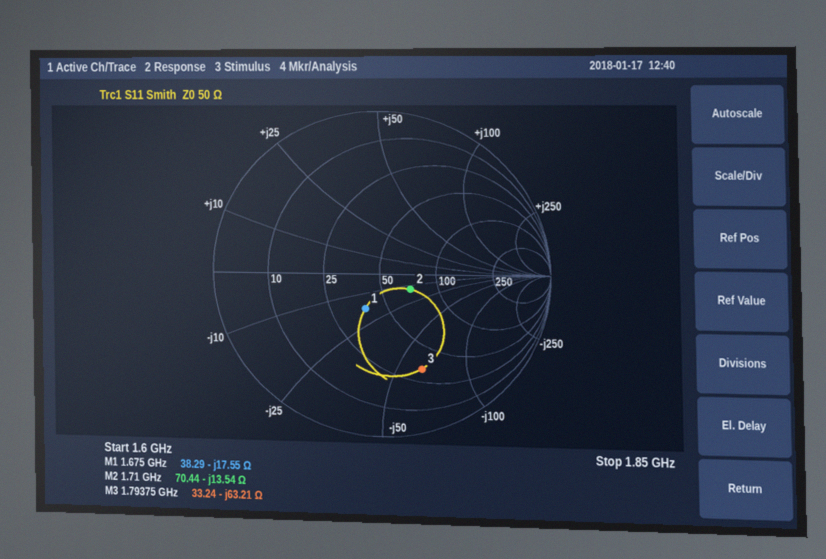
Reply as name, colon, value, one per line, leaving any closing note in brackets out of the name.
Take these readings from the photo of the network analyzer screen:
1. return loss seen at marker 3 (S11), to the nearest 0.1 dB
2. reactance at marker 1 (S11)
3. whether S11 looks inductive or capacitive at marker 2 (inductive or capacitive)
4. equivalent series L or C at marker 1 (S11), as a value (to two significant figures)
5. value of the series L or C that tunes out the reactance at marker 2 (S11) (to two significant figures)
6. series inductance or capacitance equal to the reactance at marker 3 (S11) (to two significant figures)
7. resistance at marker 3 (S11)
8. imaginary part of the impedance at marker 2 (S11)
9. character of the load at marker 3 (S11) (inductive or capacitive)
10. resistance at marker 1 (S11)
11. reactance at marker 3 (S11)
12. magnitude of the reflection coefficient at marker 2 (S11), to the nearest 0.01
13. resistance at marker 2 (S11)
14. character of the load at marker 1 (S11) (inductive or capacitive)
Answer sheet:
return loss seen at marker 3 (S11), to the nearest 0.1 dB: 4.1 dB
reactance at marker 1: -17.55 Ω
whether S11 looks inductive or capacitive at marker 2: capacitive
equivalent series L or C at marker 1 (S11), as a value: 5.4 pF
value of the series L or C that tunes out the reactance at marker 2 (S11): 1.3 nH
series inductance or capacitance equal to the reactance at marker 3 (S11): 1.4 pF
resistance at marker 3: 33.24 Ω
imaginary part of the impedance at marker 2: -13.54 Ω
character of the load at marker 3 (S11): capacitive
resistance at marker 1: 38.29 Ω
reactance at marker 3: -63.21 Ω
magnitude of the reflection coefficient at marker 2 (S11), to the nearest 0.01: 0.20
resistance at marker 2: 70.44 Ω
character of the load at marker 1 (S11): capacitive
